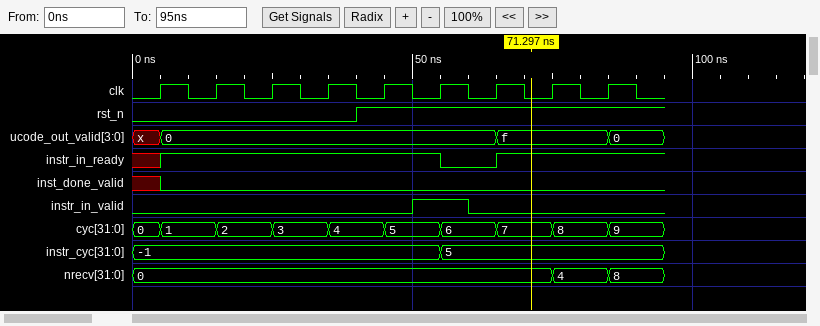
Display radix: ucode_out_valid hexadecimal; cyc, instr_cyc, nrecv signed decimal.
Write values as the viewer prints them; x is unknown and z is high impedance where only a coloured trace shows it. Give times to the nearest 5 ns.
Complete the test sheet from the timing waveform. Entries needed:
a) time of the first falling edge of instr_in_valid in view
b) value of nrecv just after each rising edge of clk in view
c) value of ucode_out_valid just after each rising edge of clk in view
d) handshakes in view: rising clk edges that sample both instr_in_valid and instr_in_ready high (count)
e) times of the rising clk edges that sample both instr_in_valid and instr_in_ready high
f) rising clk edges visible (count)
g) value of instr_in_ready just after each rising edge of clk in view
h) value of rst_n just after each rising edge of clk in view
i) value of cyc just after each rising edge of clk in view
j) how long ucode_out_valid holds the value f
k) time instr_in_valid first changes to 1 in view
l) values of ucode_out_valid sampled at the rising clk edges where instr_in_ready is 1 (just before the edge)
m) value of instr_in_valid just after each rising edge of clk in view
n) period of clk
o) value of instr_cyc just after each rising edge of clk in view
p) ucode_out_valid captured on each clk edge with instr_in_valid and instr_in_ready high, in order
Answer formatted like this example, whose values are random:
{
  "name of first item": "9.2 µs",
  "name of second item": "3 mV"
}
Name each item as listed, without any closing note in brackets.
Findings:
{
  "time of the first falling edge of instr_in_valid in view": "60 ns",
  "value of nrecv just after each rising edge of clk in view": "0, 0, 0, 0, 0, 0, 0, 4, 8",
  "value of ucode_out_valid just after each rising edge of clk in view": "0, 0, 0, 0, 0, 0, f, f, 0",
  "handshakes in view: rising clk edges that sample both instr_in_valid and instr_in_ready high": "1",
  "times of the rising clk edges that sample both instr_in_valid and instr_in_ready high": "55 ns",
  "rising clk edges visible": "9",
  "value of instr_in_ready just after each rising edge of clk in view": "1 1 1 1 1 0 1 1 1",
  "value of rst_n just after each rising edge of clk in view": "0 0 0 0 1 1 1 1 1",
  "value of cyc just after each rising edge of clk in view": "1, 2, 3, 4, 5, 6, 7, 8, 9",
  "how long ucode_out_valid holds the value f": "20 ns",
  "time instr_in_valid first changes to 1 in view": "50 ns",
  "values of ucode_out_valid sampled at the rising clk edges where instr_in_ready is 1": "0, 0, 0, 0, 0, f, f",
  "value of instr_in_valid just after each rising edge of clk in view": "0 0 0 0 0 1 0 0 0",
  "period of clk": "10 ns",
  "value of instr_cyc just after each rising edge of clk in view": "-1, -1, -1, -1, -1, 5, 5, 5, 5",
  "ucode_out_valid captured on each clk edge with instr_in_valid and instr_in_ready high, in order": "0"
}
